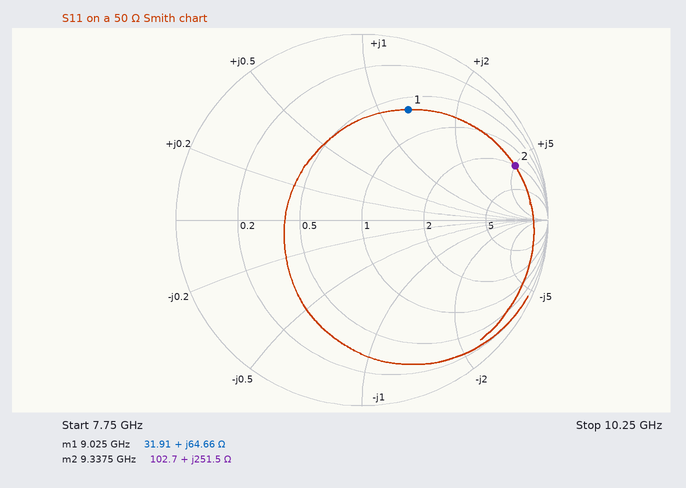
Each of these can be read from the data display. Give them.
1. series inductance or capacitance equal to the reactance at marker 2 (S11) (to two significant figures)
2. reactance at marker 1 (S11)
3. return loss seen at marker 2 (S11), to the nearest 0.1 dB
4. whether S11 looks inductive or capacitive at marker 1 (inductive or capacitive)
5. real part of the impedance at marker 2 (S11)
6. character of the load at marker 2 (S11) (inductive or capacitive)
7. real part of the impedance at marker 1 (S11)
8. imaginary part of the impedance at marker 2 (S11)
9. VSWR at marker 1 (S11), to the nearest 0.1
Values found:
4.3 nH
+64.66 Ω
1.2 dB
inductive
102.7 Ω
inductive
31.91 Ω
+251.5 Ω
4.6
